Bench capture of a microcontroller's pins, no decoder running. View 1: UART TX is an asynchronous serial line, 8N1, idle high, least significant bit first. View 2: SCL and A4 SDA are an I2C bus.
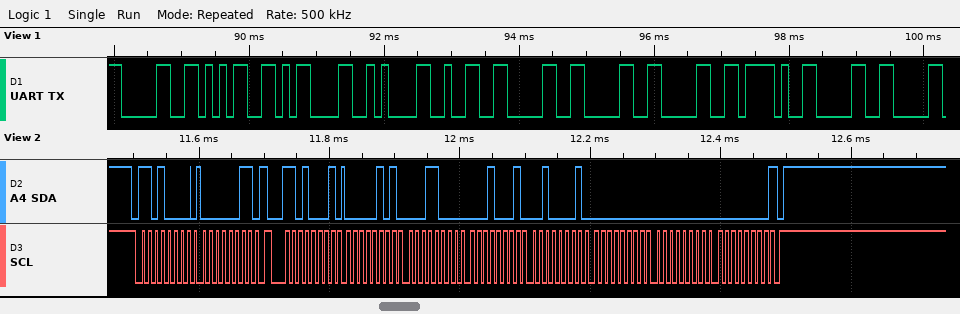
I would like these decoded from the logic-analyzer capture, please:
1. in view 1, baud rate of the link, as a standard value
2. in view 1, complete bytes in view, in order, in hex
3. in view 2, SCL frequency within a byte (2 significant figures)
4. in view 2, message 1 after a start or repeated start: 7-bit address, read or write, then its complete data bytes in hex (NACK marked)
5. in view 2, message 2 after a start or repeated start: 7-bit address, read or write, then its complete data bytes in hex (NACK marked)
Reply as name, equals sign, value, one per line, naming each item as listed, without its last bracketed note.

in view 1, baud rate of the link, as a standard value = 9600 baud
in view 1, complete bytes in view, in order, in hex = 30 35 0D 0A 32 30 30 30 2F 30
in view 2, SCL frequency within a byte = 100 kHz
in view 2, message 1 after a start or repeated start: 7-bit address, read or write, then its complete data bytes in hex = 0x68 write: 03
in view 2, message 2 after a start or repeated start: 7-bit address, read or write, then its complete data bytes in hex = 0x68 read: 05 18 11 21 00 00 00 NACK
